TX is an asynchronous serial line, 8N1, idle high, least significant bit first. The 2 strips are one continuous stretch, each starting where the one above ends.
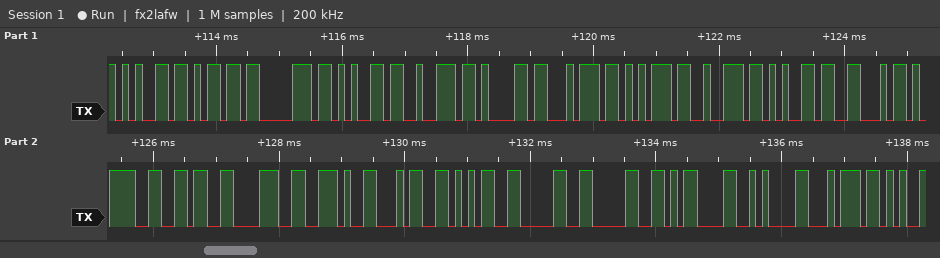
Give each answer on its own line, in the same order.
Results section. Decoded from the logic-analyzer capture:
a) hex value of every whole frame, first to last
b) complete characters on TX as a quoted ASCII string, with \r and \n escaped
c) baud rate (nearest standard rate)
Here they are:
0x65 0x6D 0x70 0x65 0x72 0x61 0x74 0x75 0x72 0x65 0x46 0x3D 0x36 0x38 0x2E 0x34 0x35 0x30 0x30 0x0D 0x0A 0x74
"emperatureF=68.4500\r\nt"
9600 baud
